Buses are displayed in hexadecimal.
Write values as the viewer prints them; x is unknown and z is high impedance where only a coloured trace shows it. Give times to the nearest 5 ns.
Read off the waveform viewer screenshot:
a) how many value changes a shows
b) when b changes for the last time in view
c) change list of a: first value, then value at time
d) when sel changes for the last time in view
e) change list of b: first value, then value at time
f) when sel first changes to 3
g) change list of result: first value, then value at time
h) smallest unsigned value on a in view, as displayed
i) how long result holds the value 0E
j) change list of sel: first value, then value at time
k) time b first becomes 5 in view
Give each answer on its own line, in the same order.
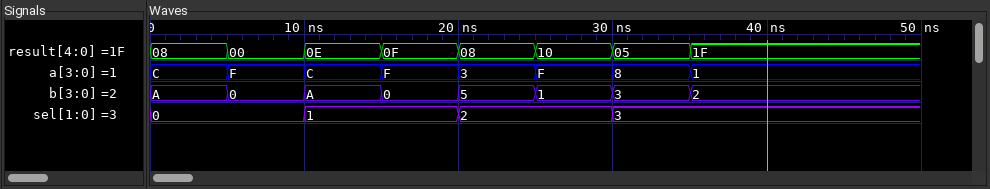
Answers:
7
35 ns
C, F at 5 ns, C at 10 ns, F at 15 ns, 3 at 20 ns, F at 25 ns, 8 at 30 ns, 1 at 35 ns
30 ns
A, 0 at 5 ns, A at 10 ns, 0 at 15 ns, 5 at 20 ns, 1 at 25 ns, 3 at 30 ns, 2 at 35 ns
30 ns
08, 00 at 5 ns, 0E at 10 ns, 0F at 15 ns, 08 at 20 ns, 10 at 25 ns, 05 at 30 ns, 1F at 35 ns
1
5 ns
0, 1 at 10 ns, 2 at 20 ns, 3 at 30 ns
20 ns
